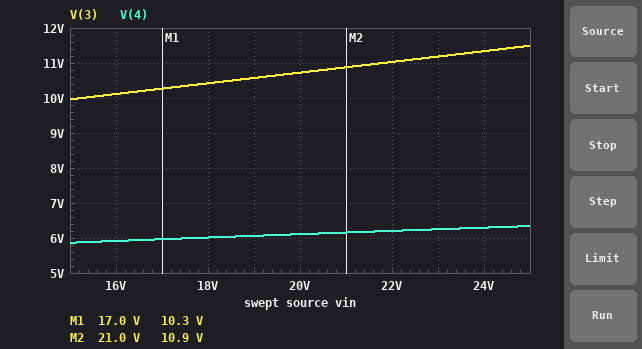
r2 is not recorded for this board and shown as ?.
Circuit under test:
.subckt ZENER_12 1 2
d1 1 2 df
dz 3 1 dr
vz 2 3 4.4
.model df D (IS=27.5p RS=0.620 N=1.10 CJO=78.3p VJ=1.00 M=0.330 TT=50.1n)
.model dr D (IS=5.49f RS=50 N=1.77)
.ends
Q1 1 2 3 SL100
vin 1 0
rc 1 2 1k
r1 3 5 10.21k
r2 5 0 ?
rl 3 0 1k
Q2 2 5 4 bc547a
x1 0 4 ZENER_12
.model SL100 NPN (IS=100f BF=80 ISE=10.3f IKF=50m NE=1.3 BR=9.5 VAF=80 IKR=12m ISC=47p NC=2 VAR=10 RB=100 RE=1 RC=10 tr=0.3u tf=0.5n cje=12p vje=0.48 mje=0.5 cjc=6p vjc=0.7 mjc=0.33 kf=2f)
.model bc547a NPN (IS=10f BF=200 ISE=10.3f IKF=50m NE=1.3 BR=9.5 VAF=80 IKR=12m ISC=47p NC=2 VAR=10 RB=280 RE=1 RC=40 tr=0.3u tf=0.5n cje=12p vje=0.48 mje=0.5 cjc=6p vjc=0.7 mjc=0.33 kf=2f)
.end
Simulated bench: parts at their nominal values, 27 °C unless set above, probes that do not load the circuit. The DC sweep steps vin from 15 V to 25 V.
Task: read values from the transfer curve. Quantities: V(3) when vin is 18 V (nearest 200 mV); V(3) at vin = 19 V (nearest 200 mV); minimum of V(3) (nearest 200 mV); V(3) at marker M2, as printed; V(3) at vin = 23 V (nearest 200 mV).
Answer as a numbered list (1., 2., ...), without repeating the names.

1. 10.4 V
2. 10.6 V
3. 10.0 V
4. 10.9 V
5. 11.2 V
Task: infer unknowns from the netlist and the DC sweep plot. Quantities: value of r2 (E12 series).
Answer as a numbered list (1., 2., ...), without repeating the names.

1. 22 kΩ
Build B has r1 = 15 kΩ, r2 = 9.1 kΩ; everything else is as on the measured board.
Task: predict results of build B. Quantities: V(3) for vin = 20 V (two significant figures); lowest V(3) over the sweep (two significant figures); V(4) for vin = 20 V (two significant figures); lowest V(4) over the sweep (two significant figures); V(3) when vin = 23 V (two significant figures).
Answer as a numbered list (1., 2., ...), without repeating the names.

1. 17 V
2. 14 V
3. 5.7 V
4. 5.0 V
5. 18 V
